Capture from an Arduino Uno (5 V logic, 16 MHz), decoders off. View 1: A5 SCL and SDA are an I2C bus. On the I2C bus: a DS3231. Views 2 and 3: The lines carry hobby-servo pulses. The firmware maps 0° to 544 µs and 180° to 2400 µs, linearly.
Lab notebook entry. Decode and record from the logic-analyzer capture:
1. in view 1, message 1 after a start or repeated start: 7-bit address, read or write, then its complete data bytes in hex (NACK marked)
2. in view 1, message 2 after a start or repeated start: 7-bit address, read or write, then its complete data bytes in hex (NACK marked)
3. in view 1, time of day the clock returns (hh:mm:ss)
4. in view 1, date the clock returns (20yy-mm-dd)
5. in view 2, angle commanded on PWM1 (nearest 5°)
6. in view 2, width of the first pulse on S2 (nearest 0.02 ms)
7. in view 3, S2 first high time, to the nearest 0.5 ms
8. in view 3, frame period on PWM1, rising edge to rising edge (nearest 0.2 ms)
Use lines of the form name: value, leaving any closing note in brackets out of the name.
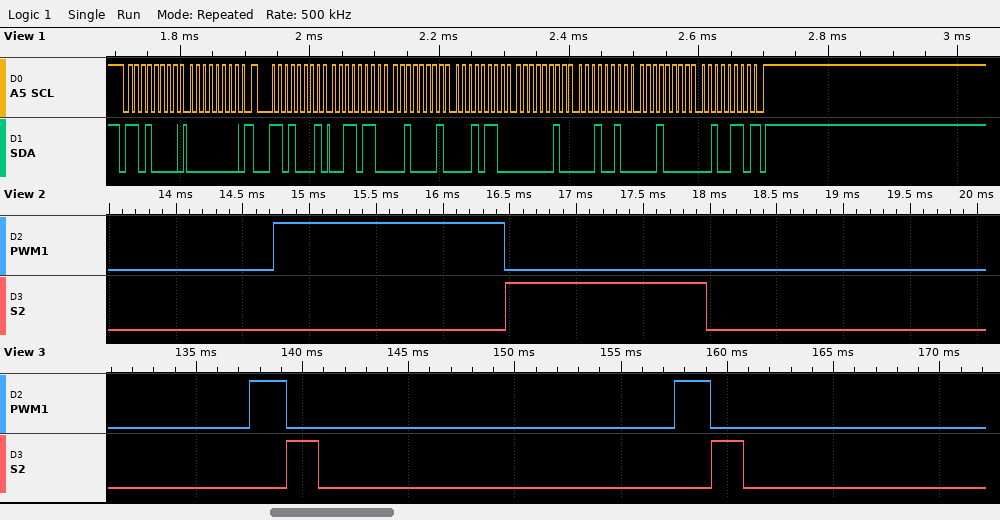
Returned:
in view 1, message 1 after a start or repeated start: 7-bit address, read or write, then its complete data bytes in hex: 0x68 write: 00
in view 1, message 2 after a start or repeated start: 7-bit address, read or write, then its complete data bytes in hex: 0x68 read: 36 21 16 02 12 10 26 NACK
in view 1, time of day the clock returns: 16:21:36
in view 1, date the clock returns: 2026-10-12
in view 2, angle commanded on PWM1: 115°
in view 2, width of the first pulse on S2: 1.50 ms
in view 3, S2 first high time, to the nearest 0.5 ms: 1.5 ms
in view 3, frame period on PWM1, rising edge to rising edge: 20.0 ms
